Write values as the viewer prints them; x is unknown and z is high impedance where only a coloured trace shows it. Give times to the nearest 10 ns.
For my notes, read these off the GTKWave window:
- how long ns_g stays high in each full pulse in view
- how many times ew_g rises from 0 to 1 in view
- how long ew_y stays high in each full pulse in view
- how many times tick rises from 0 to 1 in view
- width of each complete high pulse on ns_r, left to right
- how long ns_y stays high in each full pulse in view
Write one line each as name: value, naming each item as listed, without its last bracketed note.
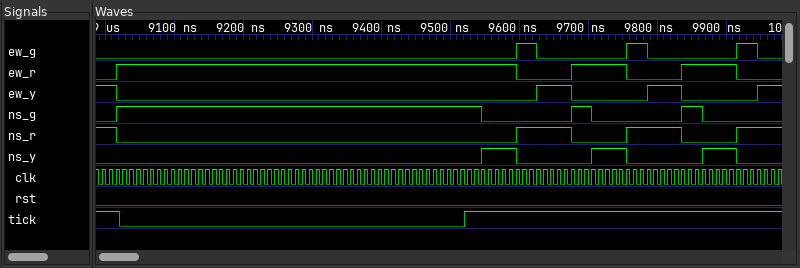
how long ns_g stays high in each full pulse in view: 530 ns, 30 ns, 30 ns
how many times ew_g rises from 0 to 1 in view: 3
how long ew_y stays high in each full pulse in view: 50 ns, 50 ns
how many times tick rises from 0 to 1 in view: 1
width of each complete high pulse on ns_r, left to right: 80 ns, 80 ns
how long ns_y stays high in each full pulse in view: 50 ns, 50 ns, 50 ns
